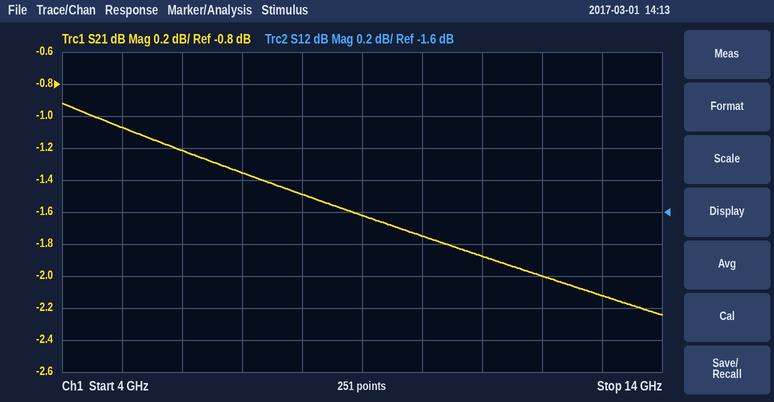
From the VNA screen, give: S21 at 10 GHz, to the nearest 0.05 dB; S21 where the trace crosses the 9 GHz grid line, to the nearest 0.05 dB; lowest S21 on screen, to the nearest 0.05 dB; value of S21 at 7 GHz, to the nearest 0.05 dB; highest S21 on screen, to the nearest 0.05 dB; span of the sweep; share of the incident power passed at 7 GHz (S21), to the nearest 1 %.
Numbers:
-1.75 dB
-1.60 dB
-2.25 dB
-1.35 dB
-0.90 dB
10 GHz
73 %
